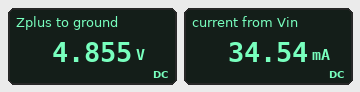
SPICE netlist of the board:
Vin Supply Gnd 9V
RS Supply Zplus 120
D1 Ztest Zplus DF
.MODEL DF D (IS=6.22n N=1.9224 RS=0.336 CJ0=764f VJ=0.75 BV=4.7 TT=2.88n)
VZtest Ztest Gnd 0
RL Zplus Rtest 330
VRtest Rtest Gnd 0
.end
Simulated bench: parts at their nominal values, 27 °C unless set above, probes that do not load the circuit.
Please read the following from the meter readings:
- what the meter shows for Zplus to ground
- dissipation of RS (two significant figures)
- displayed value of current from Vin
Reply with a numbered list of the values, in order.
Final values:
1. 4.855 V
2. 140 mW
3. 34.54 mA
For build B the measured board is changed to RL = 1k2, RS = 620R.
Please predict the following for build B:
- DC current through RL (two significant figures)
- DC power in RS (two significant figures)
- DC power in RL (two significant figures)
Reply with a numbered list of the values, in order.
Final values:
1. 4.0 mA
2. 29 mW
3. 19 mW
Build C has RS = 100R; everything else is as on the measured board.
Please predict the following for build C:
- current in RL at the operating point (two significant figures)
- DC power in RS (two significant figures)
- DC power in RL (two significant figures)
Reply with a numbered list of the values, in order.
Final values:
1. 15 mA
2. 170 mW
3. 72 mW
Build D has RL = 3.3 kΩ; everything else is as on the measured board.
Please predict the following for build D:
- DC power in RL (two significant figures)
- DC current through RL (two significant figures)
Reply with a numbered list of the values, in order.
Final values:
1. 7.2 mW
2. 1.5 mA
